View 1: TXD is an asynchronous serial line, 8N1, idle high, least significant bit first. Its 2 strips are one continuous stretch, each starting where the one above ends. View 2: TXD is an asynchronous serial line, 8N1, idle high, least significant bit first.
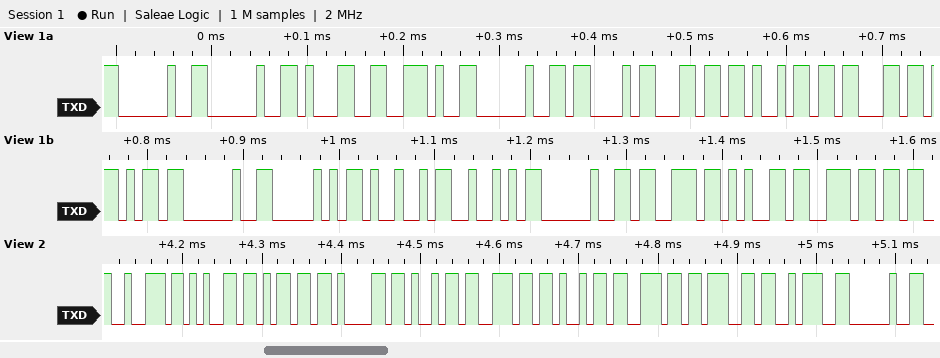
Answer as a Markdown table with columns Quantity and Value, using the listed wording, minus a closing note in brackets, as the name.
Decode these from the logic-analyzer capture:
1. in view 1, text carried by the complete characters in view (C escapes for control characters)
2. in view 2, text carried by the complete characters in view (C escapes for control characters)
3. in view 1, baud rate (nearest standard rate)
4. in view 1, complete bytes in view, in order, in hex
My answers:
| Quantity | Value |
|---|---|
| in view 1, text carried by the complete characters in view | "  1. Click PIR sen" |
| in view 2, text carried by the complete characters in view | "remaining: " |
| in view 1, baud rate | 115200 baud |
| in view 1, complete bytes in view, in order, in hex | 20 20 31 2E 20 43 6C 69 63 6B 20 50 49 52 20 73 65 6E |
